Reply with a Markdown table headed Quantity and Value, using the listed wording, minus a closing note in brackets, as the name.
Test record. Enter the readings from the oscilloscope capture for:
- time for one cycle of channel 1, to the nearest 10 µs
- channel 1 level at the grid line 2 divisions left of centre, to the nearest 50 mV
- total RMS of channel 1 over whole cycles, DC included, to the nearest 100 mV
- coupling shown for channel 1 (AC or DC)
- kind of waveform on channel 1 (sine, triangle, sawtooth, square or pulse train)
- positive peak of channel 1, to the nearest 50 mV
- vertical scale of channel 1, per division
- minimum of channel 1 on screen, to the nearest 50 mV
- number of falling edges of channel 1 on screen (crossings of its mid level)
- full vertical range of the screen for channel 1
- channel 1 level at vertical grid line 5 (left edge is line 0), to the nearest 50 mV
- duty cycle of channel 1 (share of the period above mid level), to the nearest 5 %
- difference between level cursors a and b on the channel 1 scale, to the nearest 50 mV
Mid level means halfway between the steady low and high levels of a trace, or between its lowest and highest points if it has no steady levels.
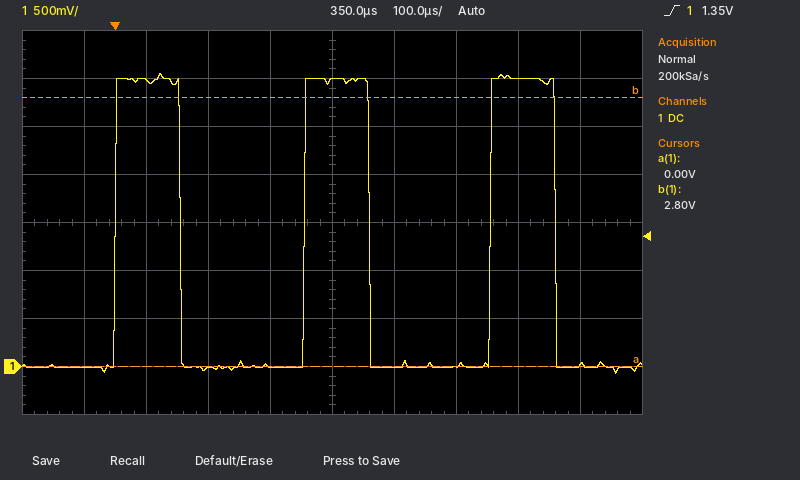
| Quantity | Value |
|---|---|
| time for one cycle of channel 1, to the nearest 10 µs | 300 µs |
| channel 1 level at the grid line 2 divisions left of centre, to the nearest 50 mV | 0 mV |
| total RMS of channel 1 over whole cycles, DC included, to the nearest 100 mV | 1.8 V |
| coupling shown for channel 1 | DC |
| kind of waveform on channel 1 | pulse train |
| positive peak of channel 1, to the nearest 50 mV | 3.05 V |
| vertical scale of channel 1, per division | 500 mV |
| minimum of channel 1 on screen, to the nearest 50 mV | -50 mV |
| number of falling edges of channel 1 on screen | 3 |
| full vertical range of the screen for channel 1 | 4 V |
| channel 1 level at vertical grid line 5 (left edge is line 0), to the nearest 50 mV | 3.00 V |
| duty cycle of channel 1 (share of the period above mid level), to the nearest 5 % | 35 % |
| difference between level cursors a and b on the channel 1 scale, to the nearest 50 mV | 2.80 V |
